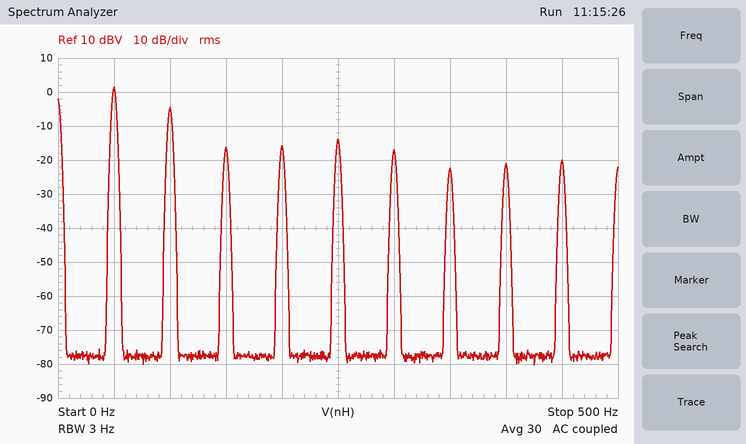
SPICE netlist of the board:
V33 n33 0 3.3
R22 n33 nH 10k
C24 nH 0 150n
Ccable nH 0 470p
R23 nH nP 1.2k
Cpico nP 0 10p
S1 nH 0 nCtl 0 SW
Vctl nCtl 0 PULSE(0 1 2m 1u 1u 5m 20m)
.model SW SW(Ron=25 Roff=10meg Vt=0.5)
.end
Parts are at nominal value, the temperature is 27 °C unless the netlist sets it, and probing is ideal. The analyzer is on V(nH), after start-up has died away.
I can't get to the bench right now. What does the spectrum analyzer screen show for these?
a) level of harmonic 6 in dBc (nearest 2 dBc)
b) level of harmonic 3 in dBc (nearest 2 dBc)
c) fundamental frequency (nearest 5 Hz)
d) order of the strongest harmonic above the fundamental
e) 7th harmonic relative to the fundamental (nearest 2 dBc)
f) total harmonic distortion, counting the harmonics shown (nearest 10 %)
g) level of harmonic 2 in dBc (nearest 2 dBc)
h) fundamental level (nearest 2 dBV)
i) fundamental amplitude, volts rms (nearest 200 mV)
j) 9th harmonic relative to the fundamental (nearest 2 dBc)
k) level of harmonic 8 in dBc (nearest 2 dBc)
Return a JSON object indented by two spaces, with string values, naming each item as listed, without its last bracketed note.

{
  "level of harmonic 6 in dBc": "-18 dBc",
  "level of harmonic 3 in dBc": "-18 dBc",
  "fundamental frequency": "50 Hz",
  "order of the strongest harmonic above the fundamental": "2",
  "7th harmonic relative to the fundamental": "-24 dBc",
  "total harmonic distortion, counting the harmonics shown": "60 %",
  "level of harmonic 2 in dBc": "-6 dBc",
  "fundamental level": "2 dBV",
  "fundamental amplitude, volts rms": "1.2 V",
  "9th harmonic relative to the fundamental": "-22 dBc",
  "level of harmonic 8 in dBc": "-22 dBc"
}
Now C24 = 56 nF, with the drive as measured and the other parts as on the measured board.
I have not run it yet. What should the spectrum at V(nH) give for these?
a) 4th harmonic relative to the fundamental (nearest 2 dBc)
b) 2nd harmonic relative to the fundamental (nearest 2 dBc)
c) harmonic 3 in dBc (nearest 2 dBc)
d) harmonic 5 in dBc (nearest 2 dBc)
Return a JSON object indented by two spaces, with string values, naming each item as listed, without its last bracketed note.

{
  "4th harmonic relative to the fundamental": "-20 dBc",
  "2nd harmonic relative to the fundamental": "-4 dBc",
  "harmonic 3 in dBc": "-14 dBc",
  "harmonic 5 in dBc": "-14 dBc"
}
